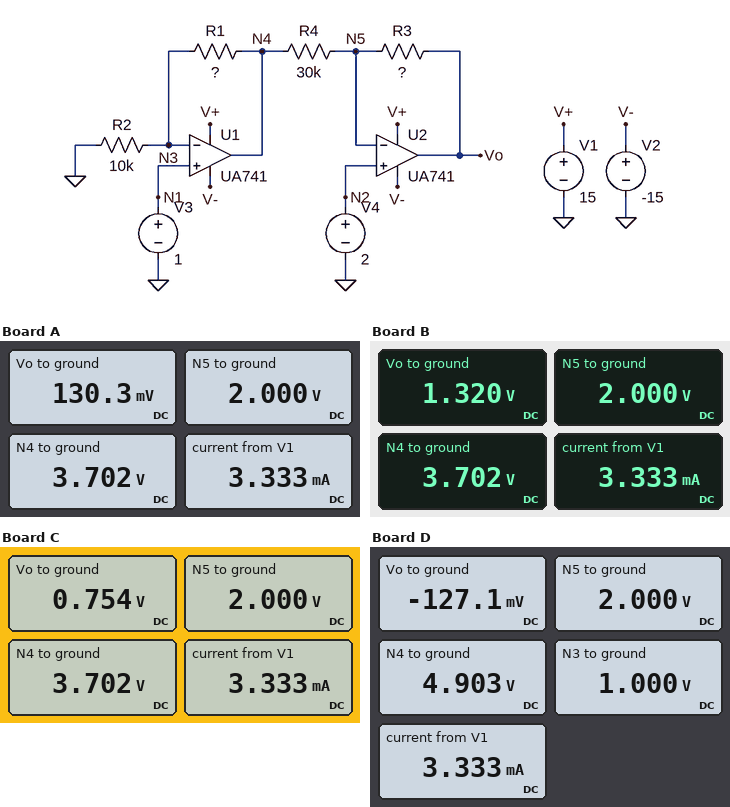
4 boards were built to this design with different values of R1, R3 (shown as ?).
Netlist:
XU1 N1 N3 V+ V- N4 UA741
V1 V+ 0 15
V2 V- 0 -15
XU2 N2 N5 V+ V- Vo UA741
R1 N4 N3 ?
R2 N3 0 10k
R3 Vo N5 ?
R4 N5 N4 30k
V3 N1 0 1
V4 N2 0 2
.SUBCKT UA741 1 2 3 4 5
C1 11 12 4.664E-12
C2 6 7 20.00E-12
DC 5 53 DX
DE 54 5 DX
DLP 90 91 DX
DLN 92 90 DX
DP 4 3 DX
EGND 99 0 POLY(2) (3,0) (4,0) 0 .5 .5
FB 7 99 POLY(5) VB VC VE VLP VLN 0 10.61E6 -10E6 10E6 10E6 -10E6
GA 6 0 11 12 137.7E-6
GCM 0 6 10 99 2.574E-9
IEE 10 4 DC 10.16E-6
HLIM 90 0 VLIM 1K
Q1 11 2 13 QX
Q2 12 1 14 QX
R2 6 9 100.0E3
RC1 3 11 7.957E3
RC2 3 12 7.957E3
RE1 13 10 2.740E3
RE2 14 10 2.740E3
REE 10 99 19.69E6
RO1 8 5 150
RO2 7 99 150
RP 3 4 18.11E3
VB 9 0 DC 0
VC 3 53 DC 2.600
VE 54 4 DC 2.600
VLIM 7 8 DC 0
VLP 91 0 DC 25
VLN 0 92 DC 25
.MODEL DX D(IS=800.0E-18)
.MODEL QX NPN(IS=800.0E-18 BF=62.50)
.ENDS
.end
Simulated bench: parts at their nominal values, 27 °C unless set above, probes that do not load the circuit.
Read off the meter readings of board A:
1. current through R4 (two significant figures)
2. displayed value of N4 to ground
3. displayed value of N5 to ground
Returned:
57 µA
3.702 V
2.000 V
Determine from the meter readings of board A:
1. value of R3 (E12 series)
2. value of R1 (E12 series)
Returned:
33 kΩ
27 kΩ
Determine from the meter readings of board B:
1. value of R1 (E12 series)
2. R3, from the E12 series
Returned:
27 kΩ
12 kΩ
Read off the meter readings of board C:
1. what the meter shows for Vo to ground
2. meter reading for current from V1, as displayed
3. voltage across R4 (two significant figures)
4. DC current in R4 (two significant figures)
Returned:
0.754 V
3.333 mA
1.7 V
57 µA
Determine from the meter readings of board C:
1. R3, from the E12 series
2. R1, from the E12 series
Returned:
22 kΩ
27 kΩ
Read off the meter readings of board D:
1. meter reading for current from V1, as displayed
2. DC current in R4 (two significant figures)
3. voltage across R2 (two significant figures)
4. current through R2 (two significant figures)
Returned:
3.333 mA
97 µA
1.0 V
100 µA
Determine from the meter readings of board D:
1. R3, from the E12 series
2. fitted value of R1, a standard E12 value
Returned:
22 kΩ
39 kΩ
